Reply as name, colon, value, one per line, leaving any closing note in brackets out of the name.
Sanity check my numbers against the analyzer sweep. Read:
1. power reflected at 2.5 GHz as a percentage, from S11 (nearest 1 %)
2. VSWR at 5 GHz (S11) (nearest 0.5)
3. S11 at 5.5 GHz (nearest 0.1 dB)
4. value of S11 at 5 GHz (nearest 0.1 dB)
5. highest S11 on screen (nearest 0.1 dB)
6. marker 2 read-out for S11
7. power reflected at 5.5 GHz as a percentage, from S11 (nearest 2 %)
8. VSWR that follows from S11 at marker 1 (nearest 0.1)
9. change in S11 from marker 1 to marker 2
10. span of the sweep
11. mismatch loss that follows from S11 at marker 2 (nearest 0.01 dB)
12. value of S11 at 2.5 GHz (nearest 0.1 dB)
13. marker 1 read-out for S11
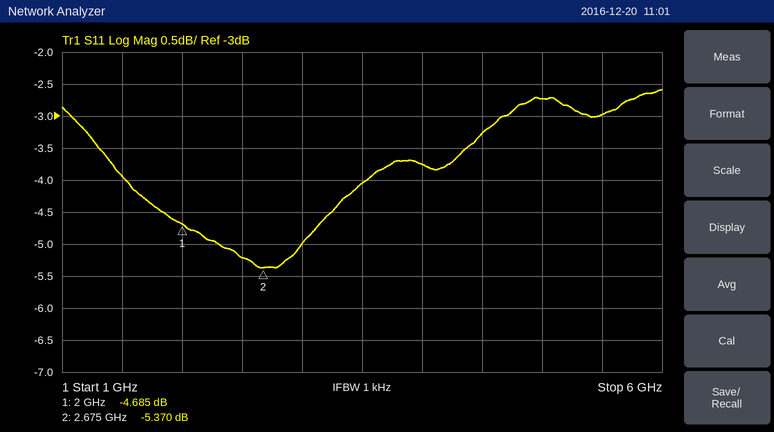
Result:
power reflected at 2.5 GHz as a percentage, from S11: 30 %
VSWR at 5 GHz (S11): 6.5
S11 at 5.5 GHz: -3.0 dB
value of S11 at 5 GHz: -2.7 dB
highest S11 on screen: -2.6 dB
marker 2 read-out for S11: -5.370 dB
power reflected at 5.5 GHz as a percentage, from S11: 50 %
VSWR that follows from S11 at marker 1: 3.8
change in S11 from marker 1 to marker 2: -0.685 dB
span of the sweep: 5 GHz
mismatch loss that follows from S11 at marker 2: 1.49 dB
value of S11 at 2.5 GHz: -5.2 dB
marker 1 read-out for S11: -4.685 dB
